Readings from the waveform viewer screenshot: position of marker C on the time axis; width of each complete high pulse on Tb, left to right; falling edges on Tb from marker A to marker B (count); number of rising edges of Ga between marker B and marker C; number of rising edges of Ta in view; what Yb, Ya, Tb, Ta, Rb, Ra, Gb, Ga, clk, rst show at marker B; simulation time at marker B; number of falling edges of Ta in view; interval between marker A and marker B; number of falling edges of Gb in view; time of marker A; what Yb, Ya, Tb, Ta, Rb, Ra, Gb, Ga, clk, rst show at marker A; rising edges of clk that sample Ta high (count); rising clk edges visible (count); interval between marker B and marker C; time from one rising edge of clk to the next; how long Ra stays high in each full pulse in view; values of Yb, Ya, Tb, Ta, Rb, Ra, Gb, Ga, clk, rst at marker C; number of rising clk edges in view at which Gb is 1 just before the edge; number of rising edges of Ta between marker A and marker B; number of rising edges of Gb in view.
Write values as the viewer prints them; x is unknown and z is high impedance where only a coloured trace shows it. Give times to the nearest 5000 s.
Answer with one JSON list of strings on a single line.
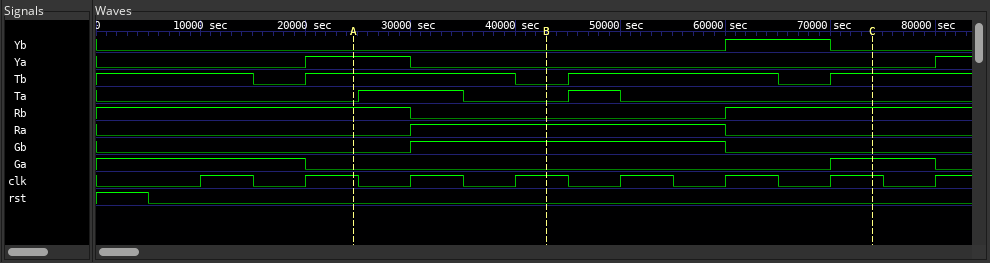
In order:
["75000 s", "20000 s, 20000 s", "1", "1", "2", "Yb=0, Ya=0, Tb=0, Ta=0, Rb=0, Ra=1, Gb=1, Ga=0, clk=1, rst=0", "45000 s", "2", "20000 s", "1", "25000 s", "Yb=0, Ya=1, Tb=1, Ta=0, Rb=1, Ra=0, Gb=0, Ga=0, clk=1, rst=0", "2", "8", "30000 s", "10000 s", "30000 s", "Yb=0, Ya=0, Tb=1, Ta=0, Rb=1, Ra=0, Gb=0, Ga=1, clk=1, rst=0", "3", "1", "1"]
